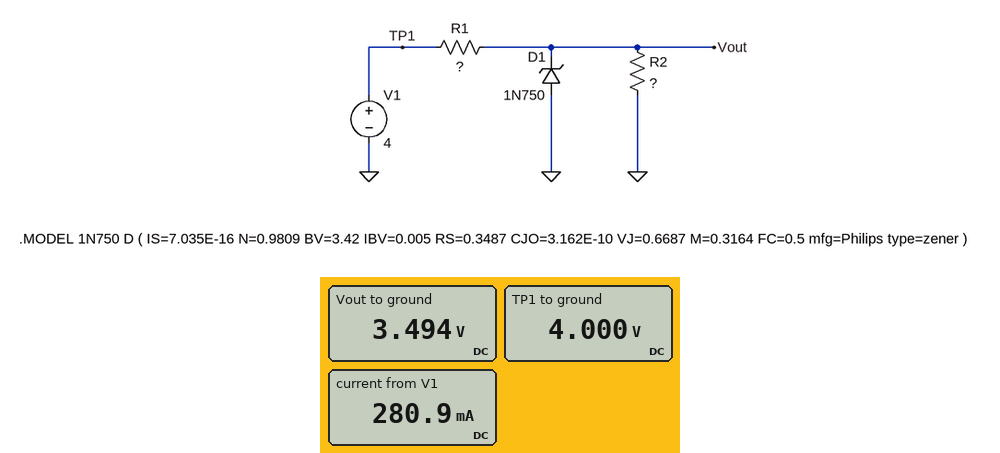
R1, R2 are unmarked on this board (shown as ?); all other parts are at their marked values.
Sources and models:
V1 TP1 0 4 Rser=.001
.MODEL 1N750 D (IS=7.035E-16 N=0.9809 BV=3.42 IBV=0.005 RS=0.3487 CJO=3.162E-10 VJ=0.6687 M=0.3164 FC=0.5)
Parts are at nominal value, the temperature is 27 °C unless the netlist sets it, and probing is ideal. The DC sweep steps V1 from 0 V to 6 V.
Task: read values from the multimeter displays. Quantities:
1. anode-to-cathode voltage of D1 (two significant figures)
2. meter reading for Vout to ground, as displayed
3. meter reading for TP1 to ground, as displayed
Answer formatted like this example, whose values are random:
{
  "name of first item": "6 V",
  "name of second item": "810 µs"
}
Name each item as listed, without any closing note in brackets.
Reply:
{
  "anode-to-cathode voltage of D1": "-3.5 V",
  "meter reading for Vout to ground, as displayed": "3.494 V",
  "meter reading for TP1 to ground, as displayed": "4.000 V"
}
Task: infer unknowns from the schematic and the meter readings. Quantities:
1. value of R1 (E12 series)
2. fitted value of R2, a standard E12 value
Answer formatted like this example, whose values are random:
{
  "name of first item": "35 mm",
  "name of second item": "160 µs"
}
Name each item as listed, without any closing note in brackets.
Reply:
{
  "value of R1": "1.8 Ω",
  "fitted value of R2, a standard E12 value": "15 Ω"
}
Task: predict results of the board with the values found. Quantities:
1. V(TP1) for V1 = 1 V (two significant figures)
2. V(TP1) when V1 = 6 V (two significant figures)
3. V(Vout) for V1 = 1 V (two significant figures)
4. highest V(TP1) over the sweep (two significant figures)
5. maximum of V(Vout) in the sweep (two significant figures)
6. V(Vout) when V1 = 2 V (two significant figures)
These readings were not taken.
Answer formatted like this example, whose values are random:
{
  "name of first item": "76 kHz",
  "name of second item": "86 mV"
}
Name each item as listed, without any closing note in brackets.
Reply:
{
  "V(TP1) for V1 = 1 V": "1.0 V",
  "V(TP1) when V1 = 6 V": "6.0 V",
  "V(Vout) for V1 = 1 V": "890 mV",
  "highest V(TP1) over the sweep": "6.0 V",
  "maximum of V(Vout) in the sweep": "3.9 V",
  "V(Vout) when V1 = 2 V": "1.8 V"
}
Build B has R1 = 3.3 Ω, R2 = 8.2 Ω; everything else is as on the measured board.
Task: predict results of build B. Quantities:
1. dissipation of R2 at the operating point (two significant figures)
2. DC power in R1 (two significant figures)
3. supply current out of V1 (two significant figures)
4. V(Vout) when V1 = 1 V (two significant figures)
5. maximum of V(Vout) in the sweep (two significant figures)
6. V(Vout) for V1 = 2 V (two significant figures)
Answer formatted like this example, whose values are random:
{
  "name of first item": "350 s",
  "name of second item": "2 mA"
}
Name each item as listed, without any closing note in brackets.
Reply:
{
  "dissipation of R2 at the operating point": "990 mW",
  "DC power in R1": "400 mW",
  "supply current out of V1": "350 mA",
  "V(Vout) when V1 = 1 V": "710 mV",
  "maximum of V(Vout) in the sweep": "3.6 V",
  "V(Vout) for V1 = 2 V": "1.4 V"
}
